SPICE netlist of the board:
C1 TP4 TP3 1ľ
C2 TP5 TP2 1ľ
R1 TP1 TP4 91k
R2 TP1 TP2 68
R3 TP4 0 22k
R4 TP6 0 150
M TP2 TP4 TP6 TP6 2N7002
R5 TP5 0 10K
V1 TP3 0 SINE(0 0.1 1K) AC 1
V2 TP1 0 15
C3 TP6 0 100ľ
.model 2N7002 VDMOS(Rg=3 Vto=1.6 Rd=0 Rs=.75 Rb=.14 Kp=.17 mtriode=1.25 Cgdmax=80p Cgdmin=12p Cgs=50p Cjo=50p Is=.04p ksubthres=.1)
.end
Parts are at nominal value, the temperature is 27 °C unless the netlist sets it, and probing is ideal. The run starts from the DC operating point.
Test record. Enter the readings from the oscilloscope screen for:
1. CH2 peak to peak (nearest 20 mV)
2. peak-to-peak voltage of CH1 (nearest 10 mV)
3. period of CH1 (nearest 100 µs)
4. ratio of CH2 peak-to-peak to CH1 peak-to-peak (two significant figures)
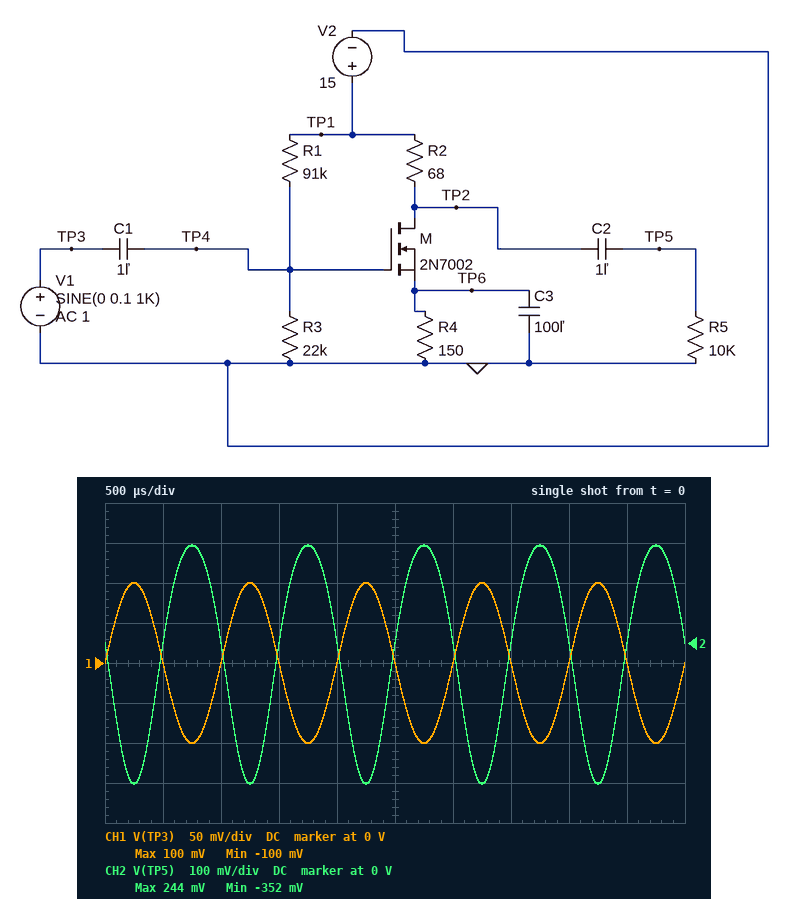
600 mV
200 mV
1.0 ms
3.0
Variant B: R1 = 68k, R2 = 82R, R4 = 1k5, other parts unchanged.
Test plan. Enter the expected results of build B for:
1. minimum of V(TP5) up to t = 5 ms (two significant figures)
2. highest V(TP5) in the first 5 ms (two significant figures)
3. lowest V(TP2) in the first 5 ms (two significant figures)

-180 mV
78 mV
15 V
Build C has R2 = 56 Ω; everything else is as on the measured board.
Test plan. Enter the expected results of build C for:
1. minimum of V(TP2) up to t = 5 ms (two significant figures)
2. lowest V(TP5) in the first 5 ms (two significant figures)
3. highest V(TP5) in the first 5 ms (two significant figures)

14 V
-290 mV
200 mV
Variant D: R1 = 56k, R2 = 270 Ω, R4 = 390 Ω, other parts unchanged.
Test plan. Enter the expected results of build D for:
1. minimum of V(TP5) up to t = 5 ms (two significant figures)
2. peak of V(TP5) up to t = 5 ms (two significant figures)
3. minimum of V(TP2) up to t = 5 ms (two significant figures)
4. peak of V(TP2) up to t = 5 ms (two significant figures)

-1.3 V
870 mV
12 V
14 V
